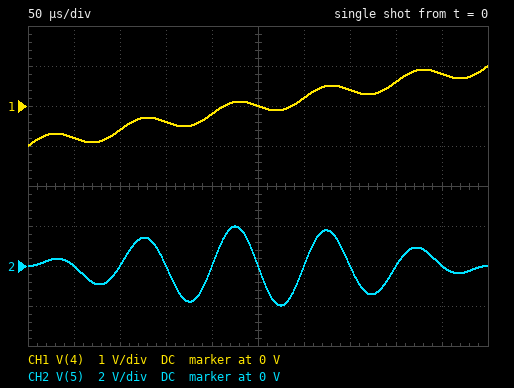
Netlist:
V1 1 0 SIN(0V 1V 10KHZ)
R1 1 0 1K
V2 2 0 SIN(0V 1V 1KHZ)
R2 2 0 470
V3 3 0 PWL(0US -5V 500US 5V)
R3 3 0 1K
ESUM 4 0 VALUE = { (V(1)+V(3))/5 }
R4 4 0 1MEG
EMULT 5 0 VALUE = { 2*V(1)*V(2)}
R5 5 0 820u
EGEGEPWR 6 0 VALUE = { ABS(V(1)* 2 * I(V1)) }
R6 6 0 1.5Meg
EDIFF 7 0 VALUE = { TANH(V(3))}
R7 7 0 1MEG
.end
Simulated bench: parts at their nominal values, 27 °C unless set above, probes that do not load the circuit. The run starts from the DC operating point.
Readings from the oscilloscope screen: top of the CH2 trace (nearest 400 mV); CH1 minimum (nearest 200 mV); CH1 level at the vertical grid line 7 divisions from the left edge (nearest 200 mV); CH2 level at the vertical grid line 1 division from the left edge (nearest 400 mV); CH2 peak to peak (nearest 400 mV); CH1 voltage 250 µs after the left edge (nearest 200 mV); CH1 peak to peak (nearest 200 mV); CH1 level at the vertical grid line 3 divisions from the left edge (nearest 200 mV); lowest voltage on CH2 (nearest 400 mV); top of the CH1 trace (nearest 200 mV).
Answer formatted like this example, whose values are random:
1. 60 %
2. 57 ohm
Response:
1. 2.0 V
2. -1.0 V
3. 400 mV
4. 0 V
5. 4.0 V
6. 0 V
7. 2.0 V
8. -400 mV
9. -2.0 V
10. 1.0 V
